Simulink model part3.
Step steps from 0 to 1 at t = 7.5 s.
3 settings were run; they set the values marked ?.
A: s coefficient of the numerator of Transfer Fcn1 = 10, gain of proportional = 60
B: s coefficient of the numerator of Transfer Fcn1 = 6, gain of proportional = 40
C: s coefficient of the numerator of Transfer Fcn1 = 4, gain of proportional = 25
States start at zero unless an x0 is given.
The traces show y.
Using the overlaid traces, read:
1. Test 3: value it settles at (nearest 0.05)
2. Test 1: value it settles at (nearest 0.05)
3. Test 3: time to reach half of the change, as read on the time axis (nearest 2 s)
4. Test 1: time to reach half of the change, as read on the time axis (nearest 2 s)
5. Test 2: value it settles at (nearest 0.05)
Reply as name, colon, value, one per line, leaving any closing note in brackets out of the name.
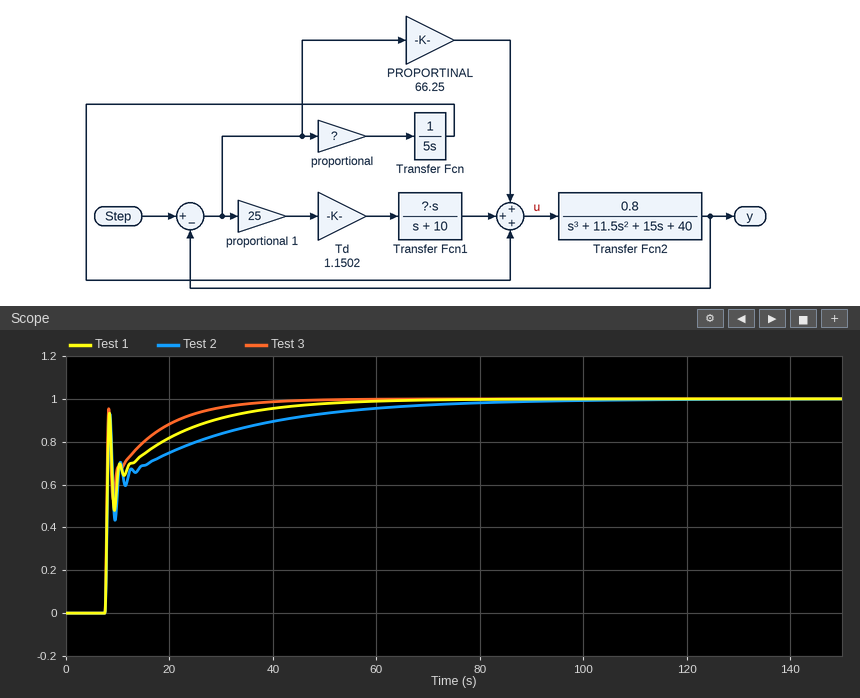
Test 3: value it settles at: 1.00
Test 1: value it settles at: 1.00
Test 3: time to reach half of the change, as read on the time axis: 8 s
Test 1: time to reach half of the change, as read on the time axis: 8 s
Test 2: value it settles at: 1.00
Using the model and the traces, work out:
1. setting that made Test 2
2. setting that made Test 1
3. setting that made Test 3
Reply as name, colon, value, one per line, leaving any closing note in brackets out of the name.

setting that made Test 2: C
setting that made Test 1: B
setting that made Test 3: A
